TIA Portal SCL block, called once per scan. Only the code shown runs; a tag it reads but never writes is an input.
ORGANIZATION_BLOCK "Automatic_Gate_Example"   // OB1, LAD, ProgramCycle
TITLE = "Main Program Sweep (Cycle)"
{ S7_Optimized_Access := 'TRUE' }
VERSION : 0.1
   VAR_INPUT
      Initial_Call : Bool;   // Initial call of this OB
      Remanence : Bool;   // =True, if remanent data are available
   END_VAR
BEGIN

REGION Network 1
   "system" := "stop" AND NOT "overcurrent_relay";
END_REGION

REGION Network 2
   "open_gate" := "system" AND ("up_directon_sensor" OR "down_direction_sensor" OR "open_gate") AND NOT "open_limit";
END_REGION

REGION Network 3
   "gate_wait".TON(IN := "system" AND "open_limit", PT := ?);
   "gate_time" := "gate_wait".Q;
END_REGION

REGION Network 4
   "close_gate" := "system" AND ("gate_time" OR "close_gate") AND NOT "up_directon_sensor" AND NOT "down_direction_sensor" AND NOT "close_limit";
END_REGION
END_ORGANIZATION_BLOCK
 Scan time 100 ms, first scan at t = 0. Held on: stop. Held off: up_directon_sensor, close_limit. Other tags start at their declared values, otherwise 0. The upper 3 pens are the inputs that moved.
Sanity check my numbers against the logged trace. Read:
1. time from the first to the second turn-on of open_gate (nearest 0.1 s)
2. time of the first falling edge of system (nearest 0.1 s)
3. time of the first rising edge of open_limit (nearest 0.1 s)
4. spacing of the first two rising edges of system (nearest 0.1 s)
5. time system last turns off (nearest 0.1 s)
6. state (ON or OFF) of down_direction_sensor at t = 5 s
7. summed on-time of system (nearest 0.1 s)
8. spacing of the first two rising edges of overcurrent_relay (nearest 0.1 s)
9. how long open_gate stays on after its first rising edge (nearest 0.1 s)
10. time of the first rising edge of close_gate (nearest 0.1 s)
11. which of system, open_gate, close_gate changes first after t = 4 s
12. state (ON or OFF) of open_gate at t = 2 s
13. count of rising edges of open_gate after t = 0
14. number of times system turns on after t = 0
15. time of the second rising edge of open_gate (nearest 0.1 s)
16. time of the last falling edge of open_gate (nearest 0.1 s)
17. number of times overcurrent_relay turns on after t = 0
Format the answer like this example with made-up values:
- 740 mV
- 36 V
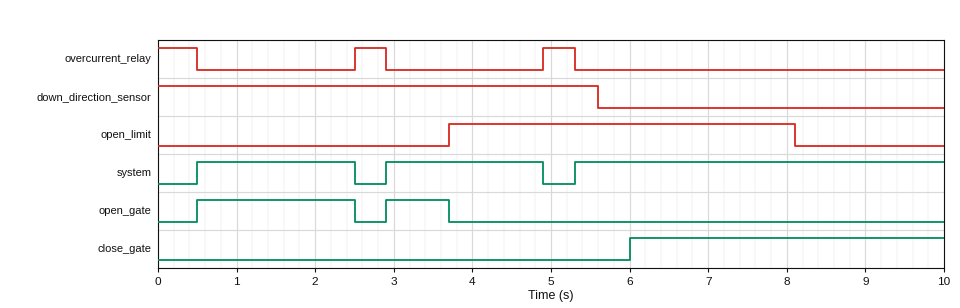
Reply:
- 2.4 s
- 2.5 s
- 3.7 s
- 2.4 s
- 4.9 s
- ON
- 8.7 s
- 2.4 s
- 2.0 s
- 6.0 s
- system
- ON
- 2
- 3
- 2.9 s
- 3.7 s
- 2
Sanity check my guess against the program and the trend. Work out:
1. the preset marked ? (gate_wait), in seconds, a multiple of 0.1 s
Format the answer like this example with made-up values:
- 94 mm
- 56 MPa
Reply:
- 0.7 s
